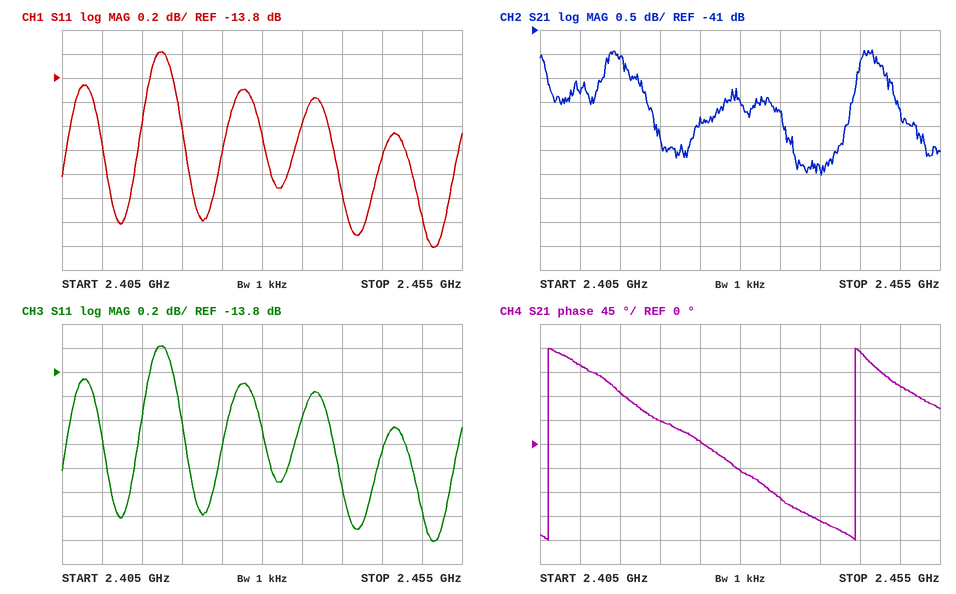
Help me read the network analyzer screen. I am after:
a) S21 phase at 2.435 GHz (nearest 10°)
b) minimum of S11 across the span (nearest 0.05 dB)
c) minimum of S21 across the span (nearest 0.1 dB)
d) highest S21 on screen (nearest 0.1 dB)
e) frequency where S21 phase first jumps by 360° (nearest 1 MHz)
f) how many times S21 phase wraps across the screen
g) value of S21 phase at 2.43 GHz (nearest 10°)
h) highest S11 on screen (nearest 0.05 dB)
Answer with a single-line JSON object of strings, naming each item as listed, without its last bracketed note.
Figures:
{"S21 phase at 2.435 GHz": "-100°", "minimum of S11 across the span": "-15.20 dB", "minimum of S21 across the span": "-44.0 dB", "highest S21 on screen": "-41.4 dB", "frequency where S21 phase first jumps by 360°": "2.406 GHz", "how many times S21 phase wraps across the screen": "2", "value of S21 phase at 2.43 GHz": "-50°", "highest S11 on screen": "-13.60 dB"}
